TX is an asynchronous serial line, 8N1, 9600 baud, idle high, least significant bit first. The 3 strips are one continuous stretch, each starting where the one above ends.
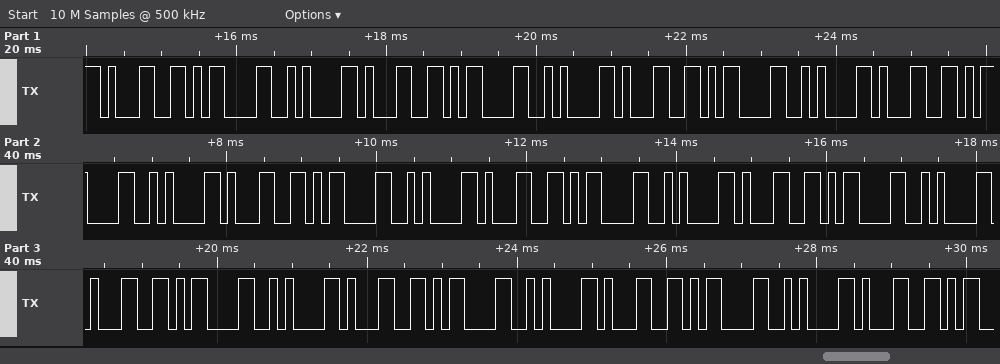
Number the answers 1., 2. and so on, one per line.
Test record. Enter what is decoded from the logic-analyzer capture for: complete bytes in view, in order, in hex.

1. 0x31 0x0D 0x0A 0x31 0x0D 0x0A 0x31 0x0D 0x0A 0x31 0x0D 0x0A 0x31 0x0D 0x0A 0x31 0x0D 0x0A 0x31 0x0D 0x0A 0x31 0x0D 0x0A 0x31 0x0D 0x0A 0x31 0x0D 0x0A 0x31
